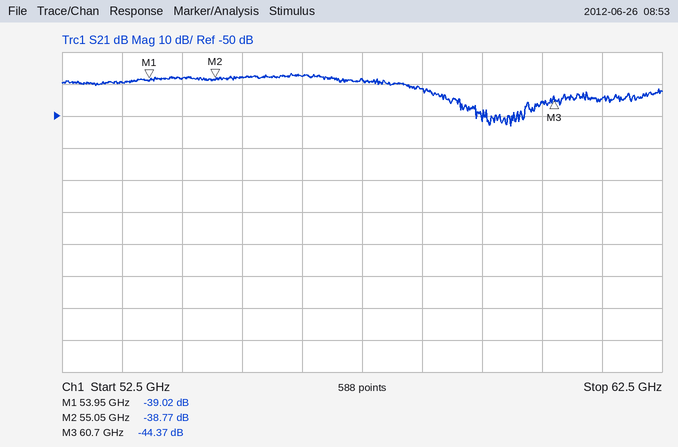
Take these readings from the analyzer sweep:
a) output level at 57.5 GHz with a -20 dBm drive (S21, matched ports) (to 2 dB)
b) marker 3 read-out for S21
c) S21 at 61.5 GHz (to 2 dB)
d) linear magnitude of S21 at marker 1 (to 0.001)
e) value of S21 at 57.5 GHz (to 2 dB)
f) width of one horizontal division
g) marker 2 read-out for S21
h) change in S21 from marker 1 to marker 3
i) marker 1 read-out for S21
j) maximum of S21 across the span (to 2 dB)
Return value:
-58 dBm
-44.37 dB
-44 dB
0.011
-38 dB
1 GHz
-38.77 dB
-5.35 dB
-39.02 dB
-36 dB
